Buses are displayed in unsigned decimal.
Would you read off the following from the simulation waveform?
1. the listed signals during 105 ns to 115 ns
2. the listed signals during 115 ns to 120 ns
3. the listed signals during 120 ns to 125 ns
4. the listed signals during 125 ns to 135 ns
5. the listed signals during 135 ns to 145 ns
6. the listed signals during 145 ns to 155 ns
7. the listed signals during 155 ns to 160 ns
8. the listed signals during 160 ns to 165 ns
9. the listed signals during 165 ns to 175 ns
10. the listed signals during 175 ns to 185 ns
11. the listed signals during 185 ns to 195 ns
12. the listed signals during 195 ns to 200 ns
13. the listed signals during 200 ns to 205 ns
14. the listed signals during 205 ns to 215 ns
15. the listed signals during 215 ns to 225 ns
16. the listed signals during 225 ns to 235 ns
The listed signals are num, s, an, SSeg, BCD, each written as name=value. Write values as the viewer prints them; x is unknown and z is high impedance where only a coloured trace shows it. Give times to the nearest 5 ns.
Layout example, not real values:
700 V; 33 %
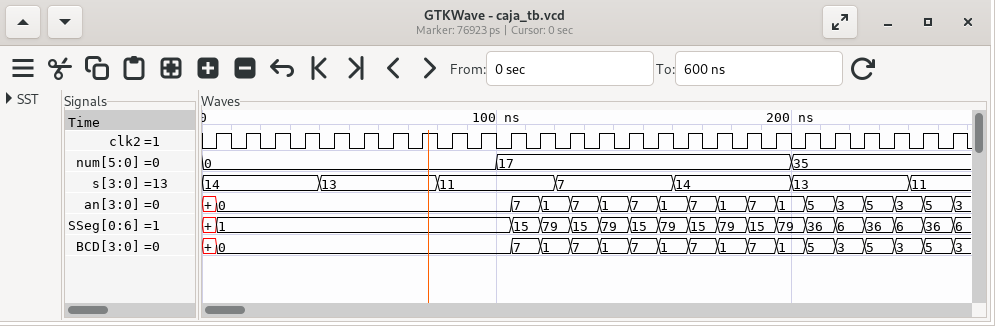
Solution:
num=17, s=11, an=7, SSeg=15, BCD=7; num=17, s=11, an=1, SSeg=79, BCD=1; num=17, s=7, an=1, SSeg=79, BCD=1; num=17, s=7, an=7, SSeg=15, BCD=7; num=17, s=7, an=1, SSeg=79, BCD=1; num=17, s=7, an=7, SSeg=15, BCD=7; num=17, s=7, an=1, SSeg=79, BCD=1; num=17, s=14, an=1, SSeg=79, BCD=1; num=17, s=14, an=7, SSeg=15, BCD=7; num=17, s=14, an=1, SSeg=79, BCD=1; num=17, s=14, an=7, SSeg=15, BCD=7; num=17, s=14, an=1, SSeg=79, BCD=1; num=35, s=13, an=1, SSeg=79, BCD=1; num=35, s=13, an=5, SSeg=36, BCD=5; num=35, s=13, an=3, SSeg=6, BCD=3; num=35, s=13, an=5, SSeg=36, BCD=5
